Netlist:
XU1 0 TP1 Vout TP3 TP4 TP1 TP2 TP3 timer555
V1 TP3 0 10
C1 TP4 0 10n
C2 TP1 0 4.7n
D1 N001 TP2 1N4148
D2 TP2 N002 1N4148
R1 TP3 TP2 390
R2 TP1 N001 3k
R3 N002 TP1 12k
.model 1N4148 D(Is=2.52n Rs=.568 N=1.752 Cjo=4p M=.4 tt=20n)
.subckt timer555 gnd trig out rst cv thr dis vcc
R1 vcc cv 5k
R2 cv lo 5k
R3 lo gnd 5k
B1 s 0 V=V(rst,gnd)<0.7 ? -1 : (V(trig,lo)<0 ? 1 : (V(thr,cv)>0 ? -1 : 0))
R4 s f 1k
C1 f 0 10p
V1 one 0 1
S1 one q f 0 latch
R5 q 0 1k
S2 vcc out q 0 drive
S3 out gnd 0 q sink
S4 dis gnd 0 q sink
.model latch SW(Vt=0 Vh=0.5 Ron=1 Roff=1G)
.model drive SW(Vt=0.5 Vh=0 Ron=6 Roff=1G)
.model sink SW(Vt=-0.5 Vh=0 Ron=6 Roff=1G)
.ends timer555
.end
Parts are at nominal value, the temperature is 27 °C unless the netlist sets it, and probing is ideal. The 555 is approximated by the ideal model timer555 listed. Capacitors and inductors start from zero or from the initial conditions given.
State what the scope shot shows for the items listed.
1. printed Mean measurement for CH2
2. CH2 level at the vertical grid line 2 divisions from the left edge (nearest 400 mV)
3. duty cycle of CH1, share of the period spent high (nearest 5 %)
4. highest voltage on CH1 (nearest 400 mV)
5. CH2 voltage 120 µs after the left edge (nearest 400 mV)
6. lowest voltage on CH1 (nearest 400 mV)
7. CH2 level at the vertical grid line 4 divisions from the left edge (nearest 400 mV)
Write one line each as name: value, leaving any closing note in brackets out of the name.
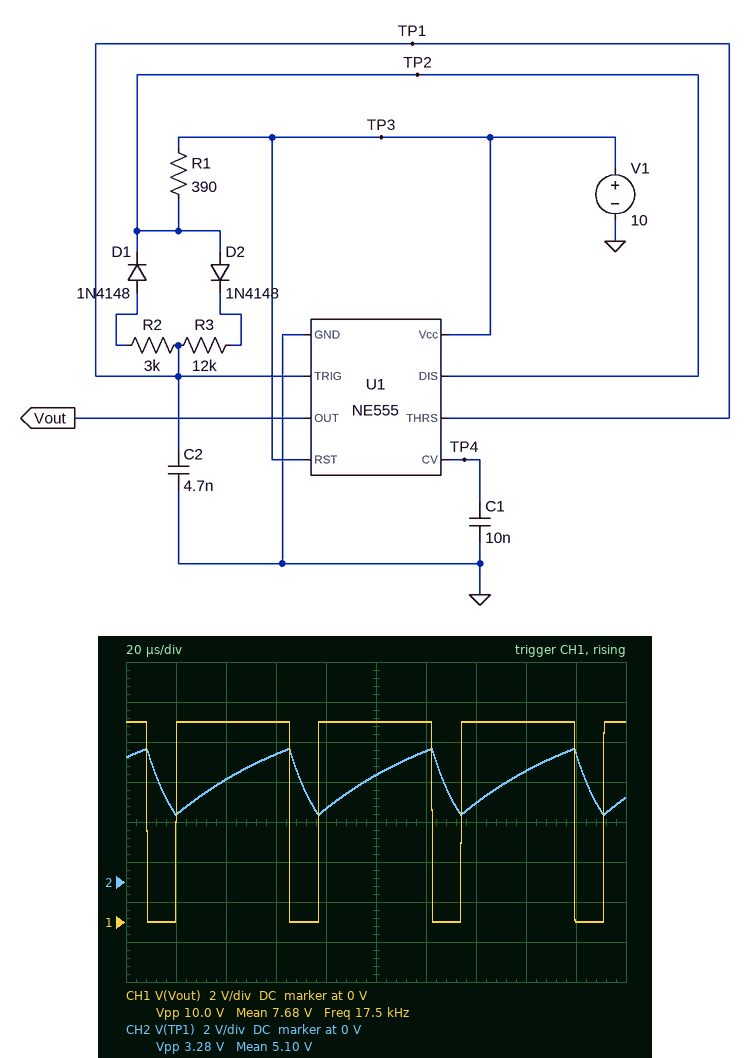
printed Mean measurement for CH2: 5.10 V
CH2 level at the vertical grid line 2 divisions from the left edge: 5.2 V
duty cycle of CH1, share of the period spent high: 80 %
highest voltage on CH1: 10.0 V
CH2 voltage 120 µs after the left edge: 6.4 V
lowest voltage on CH1: 0 V
CH2 level at the vertical grid line 4 divisions from the left edge: 3.6 V
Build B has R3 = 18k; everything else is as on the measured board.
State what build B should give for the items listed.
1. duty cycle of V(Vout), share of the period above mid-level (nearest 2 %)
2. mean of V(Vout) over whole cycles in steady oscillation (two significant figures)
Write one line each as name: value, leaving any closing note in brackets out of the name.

duty cycle of V(Vout), share of the period above mid-level: 86 %
mean of V(Vout) over whole cycles in steady oscillation: 8.5 V
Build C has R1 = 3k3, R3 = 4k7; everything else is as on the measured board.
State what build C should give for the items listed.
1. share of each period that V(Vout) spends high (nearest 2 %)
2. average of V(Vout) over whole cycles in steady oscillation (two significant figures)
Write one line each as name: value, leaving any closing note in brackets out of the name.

share of each period that V(Vout) spends high: 72 %
average of V(Vout) over whole cycles in steady oscillation: 7.2 V
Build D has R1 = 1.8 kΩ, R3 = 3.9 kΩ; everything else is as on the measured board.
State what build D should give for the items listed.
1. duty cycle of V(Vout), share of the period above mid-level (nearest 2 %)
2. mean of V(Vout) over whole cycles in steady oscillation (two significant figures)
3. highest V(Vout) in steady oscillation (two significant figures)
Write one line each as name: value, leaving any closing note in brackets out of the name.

duty cycle of V(Vout), share of the period above mid-level: 66 %
mean of V(Vout) over whole cycles in steady oscillation: 6.5 V
highest V(Vout) in steady oscillation: 10 V
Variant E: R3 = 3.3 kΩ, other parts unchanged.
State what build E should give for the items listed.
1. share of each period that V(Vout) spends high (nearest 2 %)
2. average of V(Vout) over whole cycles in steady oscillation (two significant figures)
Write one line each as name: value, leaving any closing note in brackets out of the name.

share of each period that V(Vout) spends high: 54 %
average of V(Vout) over whole cycles in steady oscillation: 5.4 V
